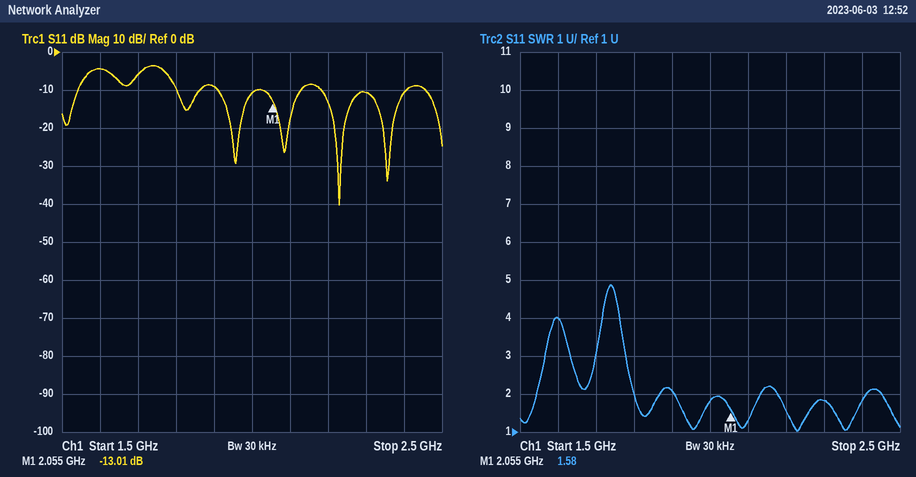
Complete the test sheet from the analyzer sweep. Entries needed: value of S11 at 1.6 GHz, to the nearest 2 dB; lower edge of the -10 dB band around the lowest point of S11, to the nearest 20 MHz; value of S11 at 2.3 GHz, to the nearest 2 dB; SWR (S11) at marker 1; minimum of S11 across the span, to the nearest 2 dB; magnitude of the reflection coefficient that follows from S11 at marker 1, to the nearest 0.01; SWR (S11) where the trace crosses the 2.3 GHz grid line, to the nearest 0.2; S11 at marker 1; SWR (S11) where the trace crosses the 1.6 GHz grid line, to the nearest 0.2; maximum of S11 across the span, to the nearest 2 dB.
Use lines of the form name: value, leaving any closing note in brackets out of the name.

value of S11 at 1.6 GHz, to the nearest 2 dB: -4 dB
lower edge of the -10 dB band around the lowest point of S11, to the nearest 20 MHz: 2.18 GHz
value of S11 at 2.3 GHz, to the nearest 2 dB: -10 dB
SWR (S11) at marker 1: 1.58
minimum of S11 across the span, to the nearest 2 dB: -40 dB
magnitude of the reflection coefficient that follows from S11 at marker 1, to the nearest 0.01: 0.22
SWR (S11) where the trace crosses the 2.3 GHz grid line, to the nearest 0.2: 1.8
S11 at marker 1: -13.01 dB
SWR (S11) where the trace crosses the 1.6 GHz grid line, to the nearest 0.2: 4.0
maximum of S11 across the span, to the nearest 2 dB: -4 dB
